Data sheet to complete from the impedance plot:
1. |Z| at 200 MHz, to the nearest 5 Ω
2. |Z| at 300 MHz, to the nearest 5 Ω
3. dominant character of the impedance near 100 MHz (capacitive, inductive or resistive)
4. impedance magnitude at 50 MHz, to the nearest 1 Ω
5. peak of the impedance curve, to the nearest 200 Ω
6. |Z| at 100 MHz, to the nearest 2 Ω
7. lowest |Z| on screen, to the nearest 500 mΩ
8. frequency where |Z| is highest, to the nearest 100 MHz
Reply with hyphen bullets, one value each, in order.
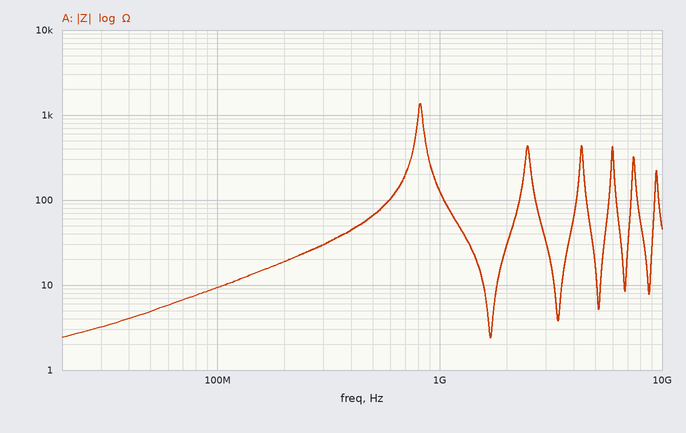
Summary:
- 20 Ω
- 30 Ω
- inductive
- 5 Ω
- 1.4 kΩ
- 10 Ω
- 2.5 Ω
- 800 MHz
